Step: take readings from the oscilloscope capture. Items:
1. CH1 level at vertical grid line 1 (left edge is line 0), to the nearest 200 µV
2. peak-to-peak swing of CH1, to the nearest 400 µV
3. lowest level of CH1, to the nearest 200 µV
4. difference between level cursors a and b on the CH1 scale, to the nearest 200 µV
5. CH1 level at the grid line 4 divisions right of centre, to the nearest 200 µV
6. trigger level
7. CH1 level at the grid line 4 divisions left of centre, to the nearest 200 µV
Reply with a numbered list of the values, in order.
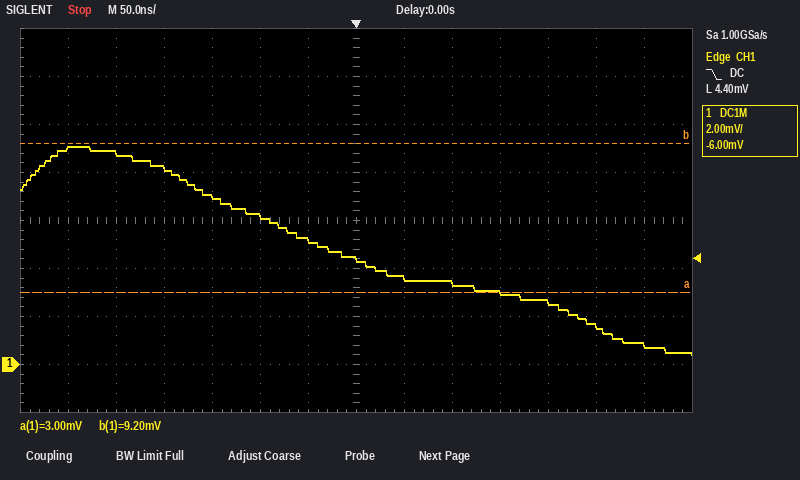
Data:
1. 9.0 mV
2. 8.8 mV
3. 400 µV
4. 6.2 mV
5. 2.6 mV
6. 4.40 mV
7. 8.2 mV
